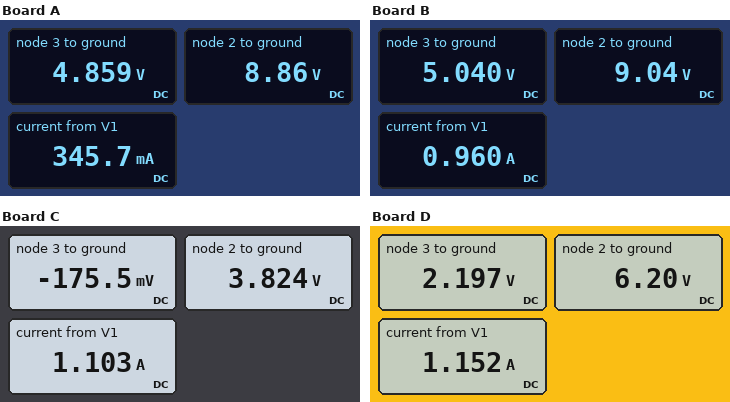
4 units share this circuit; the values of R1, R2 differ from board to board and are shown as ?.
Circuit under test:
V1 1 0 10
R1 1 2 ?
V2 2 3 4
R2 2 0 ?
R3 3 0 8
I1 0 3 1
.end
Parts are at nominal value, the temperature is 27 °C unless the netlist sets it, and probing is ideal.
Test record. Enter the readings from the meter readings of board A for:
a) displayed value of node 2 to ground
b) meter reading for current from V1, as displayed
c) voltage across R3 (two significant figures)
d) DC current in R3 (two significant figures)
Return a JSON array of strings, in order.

["8.86 V", "345.7 mA", "4.9 V", "610 mA"]
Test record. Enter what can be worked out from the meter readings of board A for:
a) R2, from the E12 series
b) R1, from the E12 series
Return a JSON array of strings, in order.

["12 Ω", "3.3 Ω"]
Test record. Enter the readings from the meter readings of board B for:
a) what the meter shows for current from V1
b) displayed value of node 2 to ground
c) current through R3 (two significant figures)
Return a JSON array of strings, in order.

["0.960 A", "9.04 V", "630 mA"]
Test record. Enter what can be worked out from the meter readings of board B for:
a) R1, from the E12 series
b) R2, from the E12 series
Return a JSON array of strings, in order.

["1 Ω", "6.8 Ω"]
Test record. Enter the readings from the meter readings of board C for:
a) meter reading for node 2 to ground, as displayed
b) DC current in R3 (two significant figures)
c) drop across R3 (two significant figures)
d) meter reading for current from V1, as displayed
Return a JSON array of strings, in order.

["3.824 V", "22 mA", "180 mV", "1.103 A"]
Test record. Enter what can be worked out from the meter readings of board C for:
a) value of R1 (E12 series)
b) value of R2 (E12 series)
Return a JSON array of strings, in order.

["5.6 Ω", "1.8 Ω"]
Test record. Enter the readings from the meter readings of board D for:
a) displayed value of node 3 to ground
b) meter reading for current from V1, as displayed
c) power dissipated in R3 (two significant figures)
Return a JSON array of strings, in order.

["2.197 V", "1.152 A", "600 mW"]
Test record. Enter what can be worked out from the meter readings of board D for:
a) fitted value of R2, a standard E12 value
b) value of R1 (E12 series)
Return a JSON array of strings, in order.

["3.3 Ω", "3.3 Ω"]
